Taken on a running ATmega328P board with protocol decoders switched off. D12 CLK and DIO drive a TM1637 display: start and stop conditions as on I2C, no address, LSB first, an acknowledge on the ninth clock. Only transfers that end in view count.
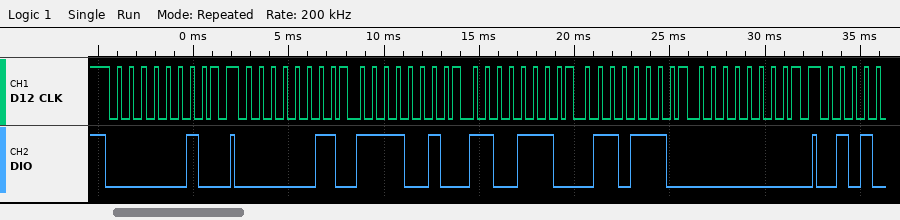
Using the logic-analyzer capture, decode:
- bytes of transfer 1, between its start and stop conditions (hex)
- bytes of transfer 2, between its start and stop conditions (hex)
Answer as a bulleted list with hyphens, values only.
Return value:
- 40
- C0 4F 73 76 00
